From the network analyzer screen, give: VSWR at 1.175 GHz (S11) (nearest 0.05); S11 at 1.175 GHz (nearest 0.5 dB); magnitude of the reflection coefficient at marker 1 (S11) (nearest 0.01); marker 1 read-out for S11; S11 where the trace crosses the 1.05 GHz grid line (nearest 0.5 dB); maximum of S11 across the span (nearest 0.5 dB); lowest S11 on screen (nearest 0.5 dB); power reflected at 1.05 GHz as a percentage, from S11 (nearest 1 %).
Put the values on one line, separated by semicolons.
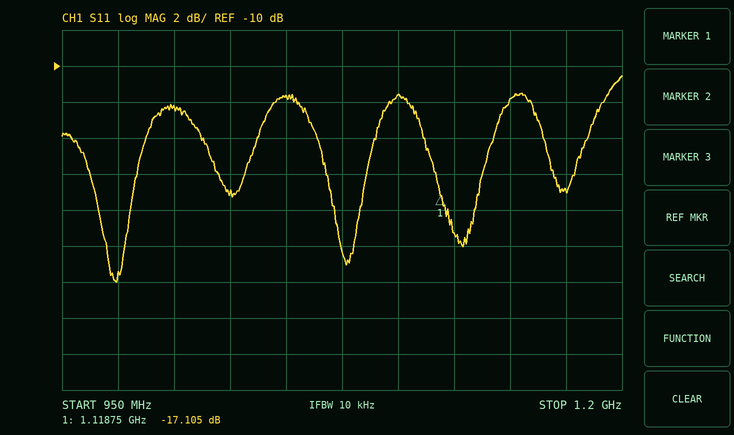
1.35; -17.0 dB; 0.14; -17.105 dB; -11.5 dB; -10.5 dB; -22.0 dB; 7 %
